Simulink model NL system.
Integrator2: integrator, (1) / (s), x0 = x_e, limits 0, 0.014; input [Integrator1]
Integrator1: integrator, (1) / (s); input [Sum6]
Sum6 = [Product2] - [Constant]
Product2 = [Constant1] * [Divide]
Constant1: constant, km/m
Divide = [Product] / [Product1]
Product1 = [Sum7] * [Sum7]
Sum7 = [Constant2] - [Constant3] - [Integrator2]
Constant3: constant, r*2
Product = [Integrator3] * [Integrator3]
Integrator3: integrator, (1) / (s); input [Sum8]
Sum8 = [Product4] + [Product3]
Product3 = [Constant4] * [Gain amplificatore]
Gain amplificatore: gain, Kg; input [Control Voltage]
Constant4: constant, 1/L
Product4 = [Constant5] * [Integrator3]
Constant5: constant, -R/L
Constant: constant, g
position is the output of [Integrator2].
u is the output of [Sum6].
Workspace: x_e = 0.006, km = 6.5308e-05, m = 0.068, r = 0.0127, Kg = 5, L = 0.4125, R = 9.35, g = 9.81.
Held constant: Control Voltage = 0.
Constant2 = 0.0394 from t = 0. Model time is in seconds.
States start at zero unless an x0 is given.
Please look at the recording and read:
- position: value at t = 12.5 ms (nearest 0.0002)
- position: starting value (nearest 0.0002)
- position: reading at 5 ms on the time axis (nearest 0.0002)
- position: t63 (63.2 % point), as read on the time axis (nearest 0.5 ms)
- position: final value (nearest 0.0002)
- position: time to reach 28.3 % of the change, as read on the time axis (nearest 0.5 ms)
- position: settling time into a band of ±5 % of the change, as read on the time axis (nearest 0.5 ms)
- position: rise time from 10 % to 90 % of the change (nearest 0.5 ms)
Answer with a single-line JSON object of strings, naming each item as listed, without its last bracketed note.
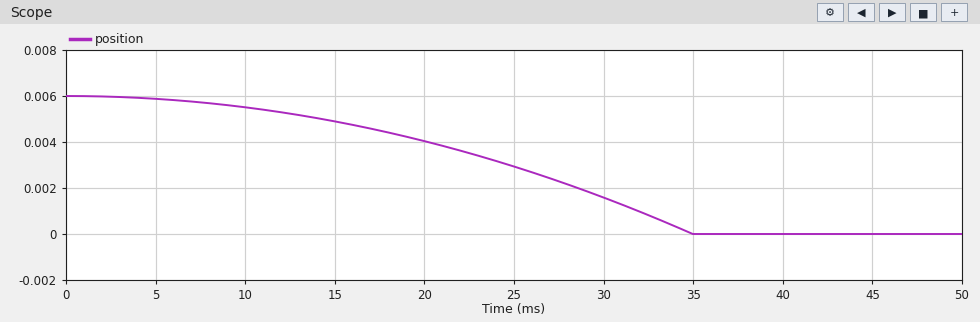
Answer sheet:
{"position: value at t = 12.5 ms": "0.0052", "position: starting value": "0.0060", "position: reading at 5 ms on the time axis": "0.0058", "position: t63 (63.2 % point), as read on the time axis": "28.0 ms", "position: final value": "0.0000", "position: time to reach 28.3 % of the change, as read on the time axis": "18.5 ms", "position: settling time into a band of ±5 % of the change, as read on the time axis": "34.0 ms", "position: rise time from 10 % to 90 % of the change": "22.0 ms"}
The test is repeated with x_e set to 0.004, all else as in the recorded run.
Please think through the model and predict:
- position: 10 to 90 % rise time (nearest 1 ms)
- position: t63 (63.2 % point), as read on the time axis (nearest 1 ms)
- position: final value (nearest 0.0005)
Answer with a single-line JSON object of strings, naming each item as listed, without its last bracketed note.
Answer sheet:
{"position: 10 to 90 % rise time": "18 ms", "position: t63 (63.2 % point), as read on the time axis": "23 ms", "position: final value": "0.0000"}
